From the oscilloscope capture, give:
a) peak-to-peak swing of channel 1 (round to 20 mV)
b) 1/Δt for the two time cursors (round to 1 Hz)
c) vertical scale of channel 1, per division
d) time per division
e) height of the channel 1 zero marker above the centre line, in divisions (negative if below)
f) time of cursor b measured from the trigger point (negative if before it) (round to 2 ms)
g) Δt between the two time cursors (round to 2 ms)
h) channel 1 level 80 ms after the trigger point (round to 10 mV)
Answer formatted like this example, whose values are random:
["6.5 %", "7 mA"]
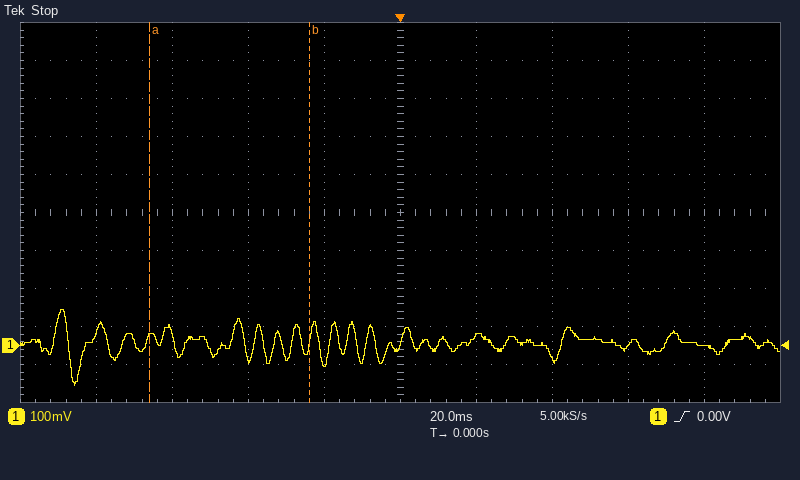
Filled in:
["200 mV", "24 Hz", "100 mV", "20 ms", "-3.5 div", "-24 ms", "42 ms", "0 mV"]
